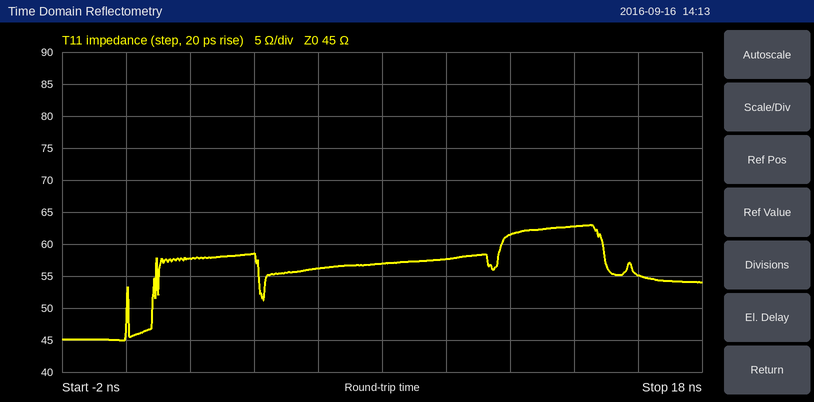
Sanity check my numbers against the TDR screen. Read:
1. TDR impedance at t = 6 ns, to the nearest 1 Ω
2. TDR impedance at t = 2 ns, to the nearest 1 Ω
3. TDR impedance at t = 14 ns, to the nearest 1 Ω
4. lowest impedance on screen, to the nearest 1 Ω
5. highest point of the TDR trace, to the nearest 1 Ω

56 Ω
58 Ω
63 Ω
45 Ω
63 Ω
